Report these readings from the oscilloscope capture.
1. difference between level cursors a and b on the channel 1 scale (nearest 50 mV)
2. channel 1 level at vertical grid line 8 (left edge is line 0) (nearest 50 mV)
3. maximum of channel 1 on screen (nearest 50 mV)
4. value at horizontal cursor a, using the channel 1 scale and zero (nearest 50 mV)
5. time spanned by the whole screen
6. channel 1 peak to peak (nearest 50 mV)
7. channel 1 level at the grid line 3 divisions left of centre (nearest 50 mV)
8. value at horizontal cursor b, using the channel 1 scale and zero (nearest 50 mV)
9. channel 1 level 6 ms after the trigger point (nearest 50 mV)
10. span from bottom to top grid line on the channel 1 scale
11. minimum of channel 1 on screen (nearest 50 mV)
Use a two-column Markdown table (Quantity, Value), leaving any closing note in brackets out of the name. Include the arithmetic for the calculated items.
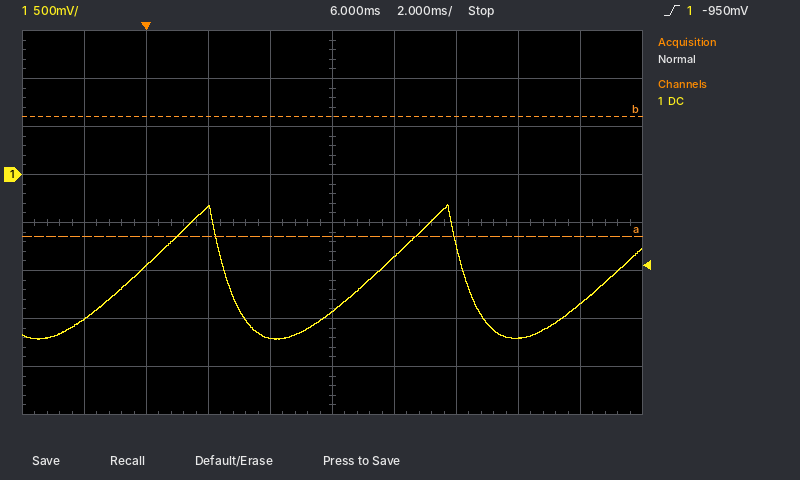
| Quantity | Value |
|---|---|
| difference between level cursors a and b on the channel 1 scale | 1.25 V |
| channel 1 level at vertical grid line 8 (left edge is line 0) | -1.70 V |
| maximum of channel 1 on screen | -300 mV |
| value at horizontal cursor a, using the channel 1 scale and zero | -650 mV |
| time spanned by the whole screen | 20 ms |
| channel 1 peak to peak | -300 mV − (-1.70 V) = 1.40 V |
| channel 1 level at the grid line 3 divisions left of centre | -950 mV |
| value at horizontal cursor b, using the channel 1 scale and zero | 600 mV |
| channel 1 level 6 ms after the trigger point | -1.45 V |
| span from bottom to top grid line on the channel 1 scale | 4 V |
| minimum of channel 1 on screen | -1.70 V |
